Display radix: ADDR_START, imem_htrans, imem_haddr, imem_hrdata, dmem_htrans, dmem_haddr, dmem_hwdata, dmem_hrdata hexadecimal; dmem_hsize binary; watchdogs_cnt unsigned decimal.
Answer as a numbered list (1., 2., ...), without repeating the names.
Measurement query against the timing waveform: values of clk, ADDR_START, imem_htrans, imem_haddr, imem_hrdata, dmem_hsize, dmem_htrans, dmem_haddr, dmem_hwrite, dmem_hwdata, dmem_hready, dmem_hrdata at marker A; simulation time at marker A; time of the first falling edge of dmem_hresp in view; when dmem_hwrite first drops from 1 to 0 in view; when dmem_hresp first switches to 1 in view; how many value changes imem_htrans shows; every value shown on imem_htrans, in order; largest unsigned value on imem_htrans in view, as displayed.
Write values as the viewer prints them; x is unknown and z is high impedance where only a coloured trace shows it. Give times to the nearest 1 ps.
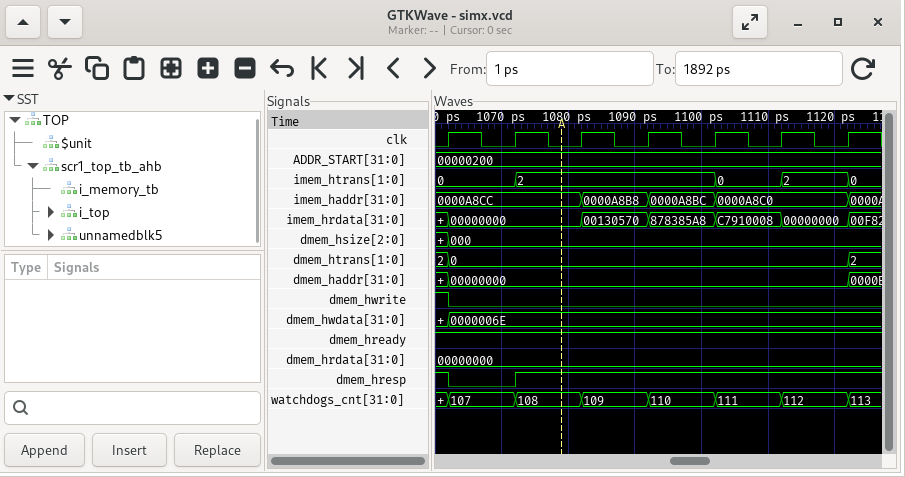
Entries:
1. clk=0, ADDR_START=00000200, imem_htrans=2, imem_haddr=0000A8CC, imem_hrdata=00000000, dmem_hsize=000, dmem_htrans=0, dmem_haddr=00000000, dmem_hwrite=0, dmem_hwdata=0000006E, dmem_hready=1, dmem_hrdata=00000000
2. 1079 ps
3. 1062 ps
4. 1062 ps
5. 1072 ps
6. 4
7. 0, 2, 0, 2, 0
8. 2
